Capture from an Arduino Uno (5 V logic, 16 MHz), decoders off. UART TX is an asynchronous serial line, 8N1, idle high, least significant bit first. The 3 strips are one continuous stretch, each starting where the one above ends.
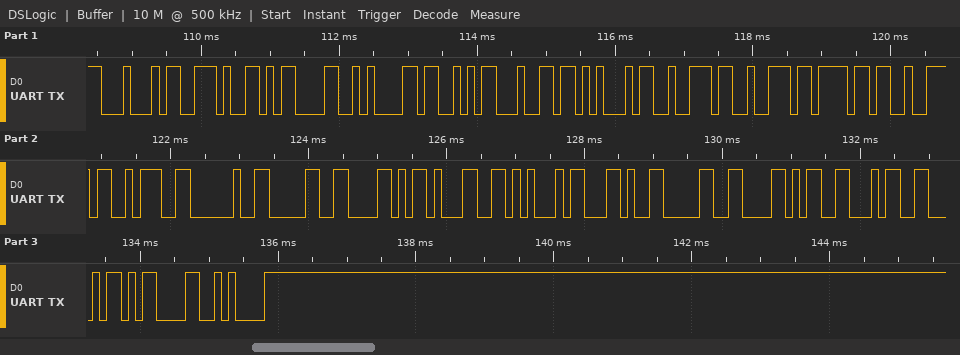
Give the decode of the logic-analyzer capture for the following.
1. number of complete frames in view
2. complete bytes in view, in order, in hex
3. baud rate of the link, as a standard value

24
0x44 0x2E 0x0D 0x0A 0x53 0x64 0x45 0x72 0x72 0x6F 0x72 0x3A 0x20 0x30 0x58 0x31 0x45 0x2C 0x30 0x58 0x46 0x46 0x0D 0x0A
9600 baud
